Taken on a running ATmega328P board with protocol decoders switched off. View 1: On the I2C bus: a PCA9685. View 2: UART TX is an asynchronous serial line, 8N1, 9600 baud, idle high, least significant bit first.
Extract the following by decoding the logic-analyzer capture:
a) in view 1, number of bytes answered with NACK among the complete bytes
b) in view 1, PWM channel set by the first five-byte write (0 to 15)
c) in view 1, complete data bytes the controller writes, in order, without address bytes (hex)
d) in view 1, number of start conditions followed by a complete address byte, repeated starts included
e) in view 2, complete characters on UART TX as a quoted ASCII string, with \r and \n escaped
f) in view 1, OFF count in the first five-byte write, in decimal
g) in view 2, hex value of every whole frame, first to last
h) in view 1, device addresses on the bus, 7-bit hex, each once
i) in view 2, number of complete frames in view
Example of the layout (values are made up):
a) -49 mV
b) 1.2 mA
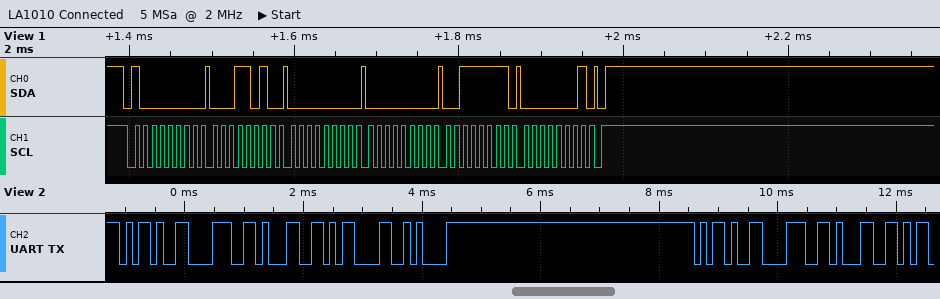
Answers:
a) 0
b) 5
c) 1A 00 00 3F 01
d) 1
e) "-81\r\n-81"
f) 319
g) 2D 38 31 0D 0A 2D 38 31
h) 0x40
i) 8
